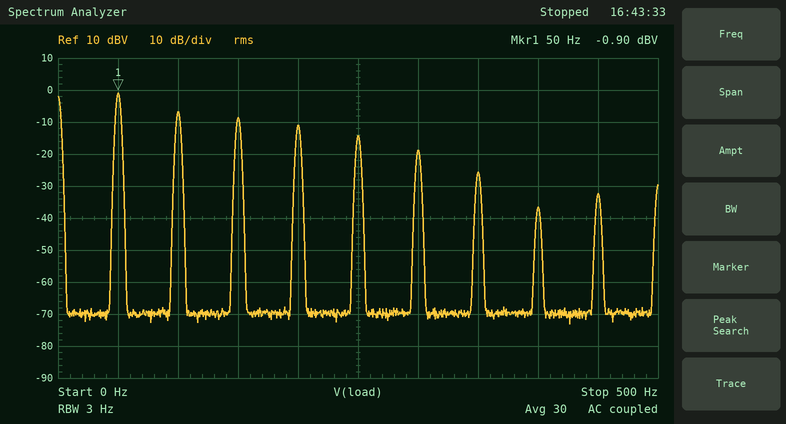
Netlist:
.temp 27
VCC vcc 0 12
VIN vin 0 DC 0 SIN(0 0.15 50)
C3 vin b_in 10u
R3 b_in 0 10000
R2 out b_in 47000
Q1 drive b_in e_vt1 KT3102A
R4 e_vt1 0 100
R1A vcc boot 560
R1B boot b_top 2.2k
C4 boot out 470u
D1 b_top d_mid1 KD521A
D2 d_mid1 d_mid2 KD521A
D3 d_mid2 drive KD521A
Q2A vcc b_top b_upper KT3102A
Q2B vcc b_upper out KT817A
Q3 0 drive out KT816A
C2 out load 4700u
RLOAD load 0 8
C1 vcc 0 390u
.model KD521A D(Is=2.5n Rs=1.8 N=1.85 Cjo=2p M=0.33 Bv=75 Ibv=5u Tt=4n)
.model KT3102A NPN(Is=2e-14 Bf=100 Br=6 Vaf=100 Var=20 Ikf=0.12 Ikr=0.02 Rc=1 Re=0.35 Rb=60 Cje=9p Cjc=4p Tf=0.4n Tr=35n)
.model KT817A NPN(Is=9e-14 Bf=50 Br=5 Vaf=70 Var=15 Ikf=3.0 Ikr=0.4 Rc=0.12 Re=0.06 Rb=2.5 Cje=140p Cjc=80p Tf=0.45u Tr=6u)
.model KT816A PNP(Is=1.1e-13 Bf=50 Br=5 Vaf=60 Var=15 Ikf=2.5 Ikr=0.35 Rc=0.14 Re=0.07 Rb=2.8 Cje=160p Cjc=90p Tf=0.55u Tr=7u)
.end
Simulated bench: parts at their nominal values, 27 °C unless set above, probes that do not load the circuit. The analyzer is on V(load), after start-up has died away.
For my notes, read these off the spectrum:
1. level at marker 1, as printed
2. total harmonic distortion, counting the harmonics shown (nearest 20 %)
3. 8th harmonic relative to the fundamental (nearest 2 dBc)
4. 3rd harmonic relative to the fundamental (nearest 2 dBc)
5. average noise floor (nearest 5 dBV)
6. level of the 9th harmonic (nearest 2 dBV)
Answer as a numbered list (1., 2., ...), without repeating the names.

1. -0.90 dBV
2. 80 %
3. -36 dBc
4. -8 dBc
5. -70 dBV
6. -32 dBV
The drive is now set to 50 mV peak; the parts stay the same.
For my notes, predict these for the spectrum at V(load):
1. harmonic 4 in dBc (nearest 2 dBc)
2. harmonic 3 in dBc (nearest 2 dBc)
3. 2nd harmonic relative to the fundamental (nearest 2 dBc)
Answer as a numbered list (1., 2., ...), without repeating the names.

1. -20 dBc
2. -16 dBc
3. -12 dBc
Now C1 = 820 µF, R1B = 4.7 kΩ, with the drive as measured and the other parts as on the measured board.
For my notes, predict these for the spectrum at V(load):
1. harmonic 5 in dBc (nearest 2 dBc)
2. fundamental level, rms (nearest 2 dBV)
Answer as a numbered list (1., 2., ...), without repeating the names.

1. -12 dBc
2. 0 dBV
